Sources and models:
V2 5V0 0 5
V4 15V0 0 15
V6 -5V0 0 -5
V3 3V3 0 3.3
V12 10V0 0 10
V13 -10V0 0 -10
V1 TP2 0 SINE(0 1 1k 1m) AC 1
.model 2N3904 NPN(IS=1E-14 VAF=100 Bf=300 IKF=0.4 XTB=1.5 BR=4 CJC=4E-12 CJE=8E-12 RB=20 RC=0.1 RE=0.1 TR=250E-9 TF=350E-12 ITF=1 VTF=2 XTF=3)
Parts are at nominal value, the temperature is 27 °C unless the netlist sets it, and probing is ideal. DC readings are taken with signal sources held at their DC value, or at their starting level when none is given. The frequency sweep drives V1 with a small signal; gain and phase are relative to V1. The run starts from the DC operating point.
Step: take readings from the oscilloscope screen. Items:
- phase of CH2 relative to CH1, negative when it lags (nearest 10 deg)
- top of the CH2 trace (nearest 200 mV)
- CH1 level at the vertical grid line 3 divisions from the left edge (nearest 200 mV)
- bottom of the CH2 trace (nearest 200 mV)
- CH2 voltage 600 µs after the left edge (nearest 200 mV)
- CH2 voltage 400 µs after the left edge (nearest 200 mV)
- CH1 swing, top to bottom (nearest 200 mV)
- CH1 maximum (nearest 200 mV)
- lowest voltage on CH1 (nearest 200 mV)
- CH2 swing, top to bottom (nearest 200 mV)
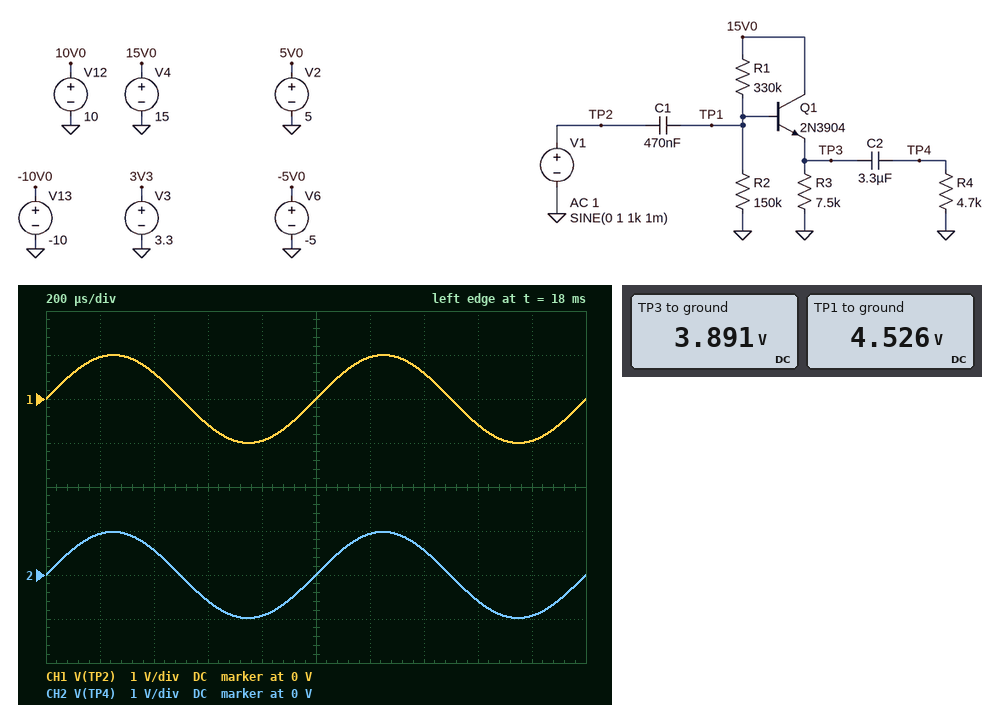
0 deg
1.0 V
-600 mV
-1.0 V
-600 mV
600 mV
2.0 V
1.0 V
-1.0 V
2.0 V
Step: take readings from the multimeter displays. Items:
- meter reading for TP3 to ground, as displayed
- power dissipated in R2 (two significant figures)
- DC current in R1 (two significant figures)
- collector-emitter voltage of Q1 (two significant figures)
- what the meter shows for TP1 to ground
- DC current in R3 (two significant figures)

3.891 V
140 µW
32 µA
11 V
4.526 V
520 µA
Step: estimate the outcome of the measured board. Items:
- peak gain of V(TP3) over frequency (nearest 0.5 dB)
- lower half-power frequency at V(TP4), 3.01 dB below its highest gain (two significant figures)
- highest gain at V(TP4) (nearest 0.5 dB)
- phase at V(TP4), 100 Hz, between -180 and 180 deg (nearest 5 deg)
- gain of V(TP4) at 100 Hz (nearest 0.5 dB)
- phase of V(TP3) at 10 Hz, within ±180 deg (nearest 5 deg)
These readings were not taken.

0 dB
11 Hz
0 dB
10 deg
0 dB
20 deg
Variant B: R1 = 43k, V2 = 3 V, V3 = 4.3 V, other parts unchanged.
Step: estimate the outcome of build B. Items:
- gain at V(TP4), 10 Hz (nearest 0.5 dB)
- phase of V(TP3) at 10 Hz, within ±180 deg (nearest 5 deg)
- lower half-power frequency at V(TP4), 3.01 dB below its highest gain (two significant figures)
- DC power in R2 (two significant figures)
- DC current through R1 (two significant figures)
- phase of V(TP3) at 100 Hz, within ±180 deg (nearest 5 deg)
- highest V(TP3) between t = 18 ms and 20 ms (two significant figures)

-6.5 dB
45 deg
16 Hz
880 µW
81 µA
5 deg
12 V
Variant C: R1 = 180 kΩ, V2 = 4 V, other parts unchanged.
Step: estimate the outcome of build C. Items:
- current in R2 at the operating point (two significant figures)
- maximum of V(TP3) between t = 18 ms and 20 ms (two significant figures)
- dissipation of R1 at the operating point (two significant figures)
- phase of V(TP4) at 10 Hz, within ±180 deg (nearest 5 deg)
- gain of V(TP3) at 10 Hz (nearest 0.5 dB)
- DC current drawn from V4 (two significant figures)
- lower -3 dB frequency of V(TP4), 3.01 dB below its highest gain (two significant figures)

44 µA
7.0 V
390 µW
70 deg
-1.0 dB
840 µA
12 Hz
